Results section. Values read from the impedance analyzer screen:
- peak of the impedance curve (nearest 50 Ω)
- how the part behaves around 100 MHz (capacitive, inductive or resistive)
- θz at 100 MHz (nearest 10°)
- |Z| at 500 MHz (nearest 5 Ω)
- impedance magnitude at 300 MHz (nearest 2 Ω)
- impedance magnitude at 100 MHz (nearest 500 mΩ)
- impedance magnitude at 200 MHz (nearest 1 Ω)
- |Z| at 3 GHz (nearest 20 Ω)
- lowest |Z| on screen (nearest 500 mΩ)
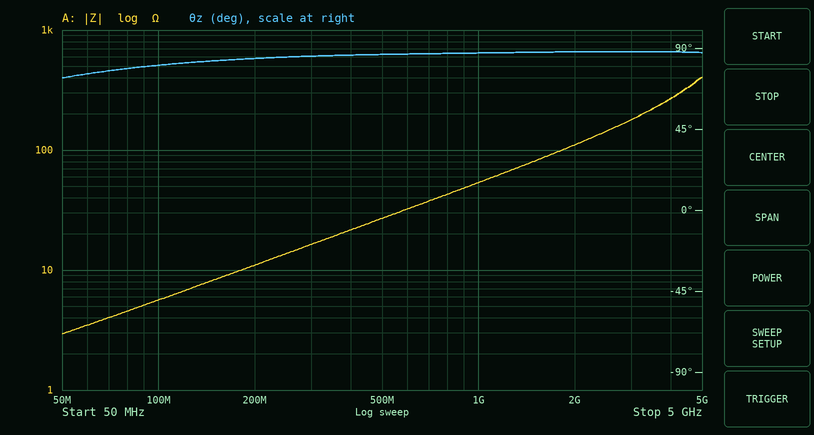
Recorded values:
400 Ω
inductive
80°
25 Ω
16 Ω
5.5 Ω
11 Ω
180 Ω
3.0 Ω
